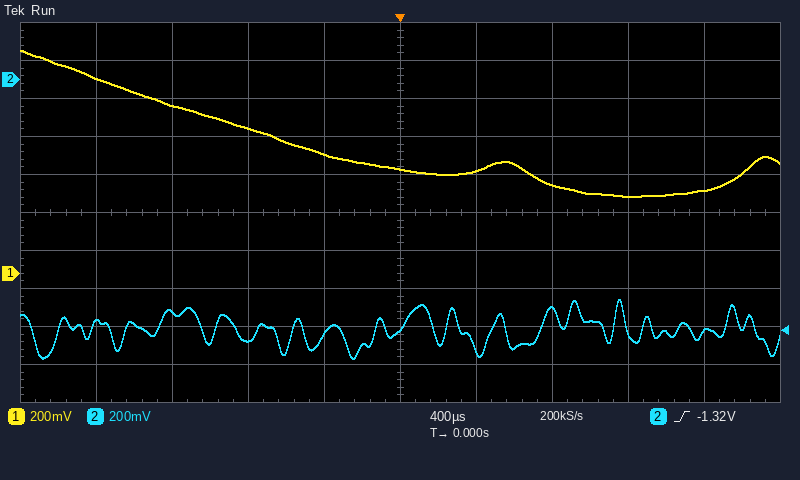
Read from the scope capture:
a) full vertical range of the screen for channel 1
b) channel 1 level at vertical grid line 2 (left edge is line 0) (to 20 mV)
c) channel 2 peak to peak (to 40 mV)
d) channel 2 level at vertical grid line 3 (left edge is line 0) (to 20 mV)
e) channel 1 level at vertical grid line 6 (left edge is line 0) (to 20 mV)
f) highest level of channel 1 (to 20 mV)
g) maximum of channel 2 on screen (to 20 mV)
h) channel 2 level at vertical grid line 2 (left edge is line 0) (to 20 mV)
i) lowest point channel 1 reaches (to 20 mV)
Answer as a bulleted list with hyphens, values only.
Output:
- 2 V
- 880 mV
- 320 mV
- -1.38 V
- 540 mV
- 1.18 V
- -1.16 V
- -1.22 V
- 400 mV
